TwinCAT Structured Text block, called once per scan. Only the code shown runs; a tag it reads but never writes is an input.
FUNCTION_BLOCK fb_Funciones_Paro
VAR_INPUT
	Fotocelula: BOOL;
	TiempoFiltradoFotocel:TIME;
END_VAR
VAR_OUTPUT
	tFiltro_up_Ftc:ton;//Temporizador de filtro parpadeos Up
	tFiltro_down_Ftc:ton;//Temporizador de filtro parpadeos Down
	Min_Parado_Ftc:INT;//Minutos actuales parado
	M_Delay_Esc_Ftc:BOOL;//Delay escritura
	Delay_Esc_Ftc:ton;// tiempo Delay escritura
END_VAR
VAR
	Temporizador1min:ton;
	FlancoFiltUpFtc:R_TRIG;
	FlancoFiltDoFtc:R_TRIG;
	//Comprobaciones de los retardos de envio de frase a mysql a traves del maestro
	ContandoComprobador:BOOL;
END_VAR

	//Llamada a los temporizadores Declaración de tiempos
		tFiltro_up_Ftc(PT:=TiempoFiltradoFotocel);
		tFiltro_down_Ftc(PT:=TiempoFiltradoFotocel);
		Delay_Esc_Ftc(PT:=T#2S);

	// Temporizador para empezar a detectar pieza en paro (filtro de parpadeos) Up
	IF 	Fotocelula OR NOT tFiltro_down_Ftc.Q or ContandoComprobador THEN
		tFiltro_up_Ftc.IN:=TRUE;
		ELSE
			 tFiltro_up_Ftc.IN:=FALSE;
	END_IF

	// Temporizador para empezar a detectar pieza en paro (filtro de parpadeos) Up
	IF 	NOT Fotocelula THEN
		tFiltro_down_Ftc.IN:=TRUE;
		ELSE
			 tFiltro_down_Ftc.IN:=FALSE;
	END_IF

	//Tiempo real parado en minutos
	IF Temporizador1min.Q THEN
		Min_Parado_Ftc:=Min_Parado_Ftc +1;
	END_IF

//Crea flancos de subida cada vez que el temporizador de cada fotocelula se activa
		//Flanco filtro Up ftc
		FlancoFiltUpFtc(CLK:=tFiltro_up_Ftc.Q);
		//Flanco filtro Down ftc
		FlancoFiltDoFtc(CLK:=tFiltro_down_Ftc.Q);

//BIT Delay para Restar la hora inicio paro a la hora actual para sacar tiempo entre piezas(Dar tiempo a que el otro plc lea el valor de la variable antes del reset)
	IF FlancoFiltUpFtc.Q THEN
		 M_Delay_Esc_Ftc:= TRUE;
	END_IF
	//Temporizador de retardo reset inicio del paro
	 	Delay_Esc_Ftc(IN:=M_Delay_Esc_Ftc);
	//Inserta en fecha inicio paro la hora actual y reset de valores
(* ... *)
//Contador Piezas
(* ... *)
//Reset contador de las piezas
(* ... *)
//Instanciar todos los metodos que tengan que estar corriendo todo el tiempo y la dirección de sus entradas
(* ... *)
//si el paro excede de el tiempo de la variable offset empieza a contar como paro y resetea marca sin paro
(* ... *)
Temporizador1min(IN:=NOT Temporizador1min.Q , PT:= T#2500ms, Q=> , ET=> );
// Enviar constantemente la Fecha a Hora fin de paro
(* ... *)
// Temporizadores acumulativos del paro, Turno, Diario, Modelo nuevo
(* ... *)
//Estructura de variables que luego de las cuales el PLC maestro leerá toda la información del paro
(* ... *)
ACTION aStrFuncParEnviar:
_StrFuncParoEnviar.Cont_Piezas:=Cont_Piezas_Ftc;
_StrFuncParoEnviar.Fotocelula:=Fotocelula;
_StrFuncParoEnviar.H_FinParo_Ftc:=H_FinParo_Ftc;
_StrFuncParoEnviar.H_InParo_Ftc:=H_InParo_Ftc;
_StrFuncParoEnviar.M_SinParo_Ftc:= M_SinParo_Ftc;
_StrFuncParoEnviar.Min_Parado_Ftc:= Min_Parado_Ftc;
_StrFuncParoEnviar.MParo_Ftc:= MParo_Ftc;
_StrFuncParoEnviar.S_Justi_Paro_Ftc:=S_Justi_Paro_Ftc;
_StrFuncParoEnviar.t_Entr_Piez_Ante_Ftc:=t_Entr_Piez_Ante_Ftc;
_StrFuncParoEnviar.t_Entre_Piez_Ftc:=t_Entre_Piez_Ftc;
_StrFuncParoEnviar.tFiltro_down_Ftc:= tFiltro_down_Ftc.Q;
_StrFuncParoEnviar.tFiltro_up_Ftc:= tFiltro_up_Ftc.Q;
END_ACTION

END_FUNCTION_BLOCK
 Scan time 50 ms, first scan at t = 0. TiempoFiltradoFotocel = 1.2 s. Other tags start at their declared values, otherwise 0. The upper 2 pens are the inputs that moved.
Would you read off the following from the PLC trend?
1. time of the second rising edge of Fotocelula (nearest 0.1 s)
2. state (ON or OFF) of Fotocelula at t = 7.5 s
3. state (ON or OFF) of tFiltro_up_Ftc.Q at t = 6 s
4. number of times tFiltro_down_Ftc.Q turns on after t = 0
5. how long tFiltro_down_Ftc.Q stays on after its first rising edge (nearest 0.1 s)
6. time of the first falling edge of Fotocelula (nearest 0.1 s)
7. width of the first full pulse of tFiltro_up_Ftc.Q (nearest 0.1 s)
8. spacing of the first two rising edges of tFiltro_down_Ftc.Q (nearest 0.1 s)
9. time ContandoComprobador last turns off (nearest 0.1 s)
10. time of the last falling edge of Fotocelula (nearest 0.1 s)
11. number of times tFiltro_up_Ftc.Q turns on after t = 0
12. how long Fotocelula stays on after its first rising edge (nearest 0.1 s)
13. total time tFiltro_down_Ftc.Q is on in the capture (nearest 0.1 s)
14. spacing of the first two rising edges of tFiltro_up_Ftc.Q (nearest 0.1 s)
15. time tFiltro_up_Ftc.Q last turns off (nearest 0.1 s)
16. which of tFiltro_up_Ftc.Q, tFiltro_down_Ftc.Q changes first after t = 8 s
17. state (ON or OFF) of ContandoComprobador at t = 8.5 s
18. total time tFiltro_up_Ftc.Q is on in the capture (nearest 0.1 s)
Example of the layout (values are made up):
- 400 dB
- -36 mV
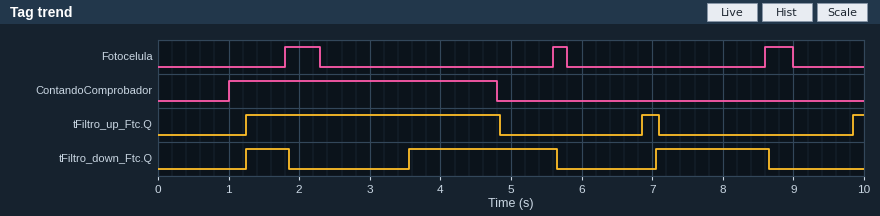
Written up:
- 5.6 s
- OFF
- OFF
- 3
- 0.6 s
- 2.3 s
- 3.6 s
- 2.3 s
- 4.8 s
- 9.0 s
- 3
- 0.5 s
- 4.3 s
- 5.6 s
- 7.1 s
- tFiltro_down_Ftc.Q
- OFF
- 4.0 s
